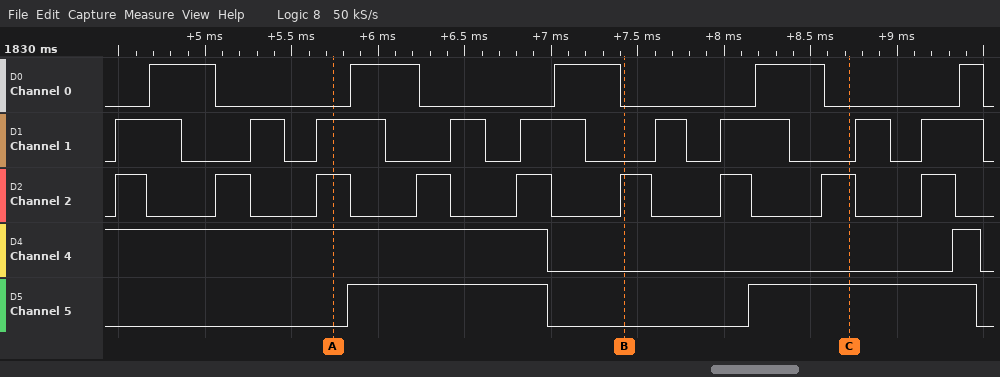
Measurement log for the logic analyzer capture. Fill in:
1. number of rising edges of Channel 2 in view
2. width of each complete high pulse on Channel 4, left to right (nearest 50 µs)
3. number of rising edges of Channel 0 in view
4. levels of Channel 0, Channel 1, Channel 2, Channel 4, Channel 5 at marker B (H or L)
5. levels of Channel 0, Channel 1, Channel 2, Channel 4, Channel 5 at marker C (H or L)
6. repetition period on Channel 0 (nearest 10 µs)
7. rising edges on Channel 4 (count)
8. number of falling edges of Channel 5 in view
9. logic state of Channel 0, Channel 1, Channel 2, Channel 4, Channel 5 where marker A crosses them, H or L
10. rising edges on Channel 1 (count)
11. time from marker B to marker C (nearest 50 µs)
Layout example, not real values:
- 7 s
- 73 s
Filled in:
- 9
- 150 µs
- 5
- Channel 0=L, Channel 1=L, Channel 2=H, Channel 4=L, Channel 5=L
- Channel 0=L, Channel 1=L, Channel 2=H, Channel 4=L, Channel 5=H
- 1170 µs
- 1
- 2
- Channel 0=L, Channel 1=H, Channel 2=H, Channel 4=H, Channel 5=L
- 9
- 1300 µs
